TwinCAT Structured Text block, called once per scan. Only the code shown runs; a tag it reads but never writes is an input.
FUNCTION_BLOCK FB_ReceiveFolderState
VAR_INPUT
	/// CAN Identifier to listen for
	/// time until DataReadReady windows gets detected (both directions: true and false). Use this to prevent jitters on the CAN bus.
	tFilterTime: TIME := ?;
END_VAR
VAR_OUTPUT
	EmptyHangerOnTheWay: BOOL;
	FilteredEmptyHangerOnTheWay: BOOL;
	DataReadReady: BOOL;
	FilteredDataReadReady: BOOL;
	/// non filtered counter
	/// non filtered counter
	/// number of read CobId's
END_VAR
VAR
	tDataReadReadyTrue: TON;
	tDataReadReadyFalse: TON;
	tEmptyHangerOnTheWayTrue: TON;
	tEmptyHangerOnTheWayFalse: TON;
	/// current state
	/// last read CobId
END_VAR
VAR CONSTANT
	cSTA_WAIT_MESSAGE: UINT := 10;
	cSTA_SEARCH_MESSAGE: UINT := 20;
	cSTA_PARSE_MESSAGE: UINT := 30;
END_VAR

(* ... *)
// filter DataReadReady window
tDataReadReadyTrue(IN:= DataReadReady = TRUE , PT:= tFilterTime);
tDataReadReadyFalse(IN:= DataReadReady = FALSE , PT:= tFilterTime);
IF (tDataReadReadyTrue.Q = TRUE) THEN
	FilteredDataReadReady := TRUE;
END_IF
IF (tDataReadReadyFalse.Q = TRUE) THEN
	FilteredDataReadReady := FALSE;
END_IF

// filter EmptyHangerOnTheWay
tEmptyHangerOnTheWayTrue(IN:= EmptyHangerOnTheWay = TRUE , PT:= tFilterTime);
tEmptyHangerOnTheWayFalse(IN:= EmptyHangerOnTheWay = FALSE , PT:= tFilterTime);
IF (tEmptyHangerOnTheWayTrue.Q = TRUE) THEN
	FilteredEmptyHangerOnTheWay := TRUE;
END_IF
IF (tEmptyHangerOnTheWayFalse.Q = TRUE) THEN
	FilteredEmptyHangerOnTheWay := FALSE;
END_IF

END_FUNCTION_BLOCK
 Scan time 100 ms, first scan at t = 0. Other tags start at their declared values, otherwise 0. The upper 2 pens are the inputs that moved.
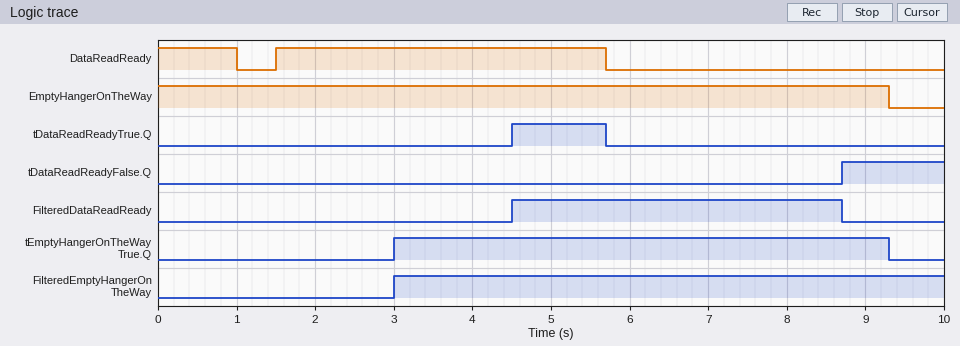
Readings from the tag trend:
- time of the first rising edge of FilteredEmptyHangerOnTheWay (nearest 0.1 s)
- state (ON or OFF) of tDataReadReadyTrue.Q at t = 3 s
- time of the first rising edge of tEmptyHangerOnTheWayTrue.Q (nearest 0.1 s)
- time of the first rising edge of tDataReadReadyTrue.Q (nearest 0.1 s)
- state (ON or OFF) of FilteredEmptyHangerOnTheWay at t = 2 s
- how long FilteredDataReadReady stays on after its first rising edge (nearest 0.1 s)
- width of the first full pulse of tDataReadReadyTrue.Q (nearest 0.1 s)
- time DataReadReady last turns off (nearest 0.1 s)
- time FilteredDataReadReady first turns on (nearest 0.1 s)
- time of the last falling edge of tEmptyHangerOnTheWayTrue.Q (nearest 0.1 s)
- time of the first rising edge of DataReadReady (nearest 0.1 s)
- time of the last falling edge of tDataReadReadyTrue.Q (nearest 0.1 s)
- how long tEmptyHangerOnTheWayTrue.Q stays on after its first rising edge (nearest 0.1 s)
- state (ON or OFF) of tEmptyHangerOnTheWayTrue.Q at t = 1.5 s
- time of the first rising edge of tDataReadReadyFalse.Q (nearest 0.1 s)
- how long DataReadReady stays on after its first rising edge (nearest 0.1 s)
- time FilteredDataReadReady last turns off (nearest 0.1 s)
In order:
3.0 s
OFF
3.0 s
4.5 s
OFF
4.2 s
1.2 s
5.7 s
4.5 s
9.3 s
1.5 s
5.7 s
6.3 s
OFF
8.7 s
4.2 s
8.7 s
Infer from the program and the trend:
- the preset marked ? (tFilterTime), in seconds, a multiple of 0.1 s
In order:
3.0 s
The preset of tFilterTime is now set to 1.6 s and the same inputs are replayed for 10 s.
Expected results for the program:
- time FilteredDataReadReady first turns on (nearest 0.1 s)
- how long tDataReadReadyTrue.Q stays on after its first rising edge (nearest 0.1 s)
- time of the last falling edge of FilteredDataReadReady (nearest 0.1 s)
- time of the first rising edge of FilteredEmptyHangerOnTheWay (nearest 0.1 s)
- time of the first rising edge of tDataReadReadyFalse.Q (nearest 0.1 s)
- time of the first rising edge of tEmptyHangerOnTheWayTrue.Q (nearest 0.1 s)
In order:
3.1 s
2.6 s
7.3 s
1.6 s
7.3 s
1.6 s
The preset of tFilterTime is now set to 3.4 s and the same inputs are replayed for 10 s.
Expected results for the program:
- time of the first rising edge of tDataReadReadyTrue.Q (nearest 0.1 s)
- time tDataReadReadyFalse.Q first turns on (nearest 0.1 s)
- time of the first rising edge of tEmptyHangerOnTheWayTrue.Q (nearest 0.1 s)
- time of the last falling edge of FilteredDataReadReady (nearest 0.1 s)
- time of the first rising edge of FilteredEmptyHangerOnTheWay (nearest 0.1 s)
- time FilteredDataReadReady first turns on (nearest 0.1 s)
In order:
4.9 s
9.1 s
3.4 s
9.1 s
3.4 s
4.9 s
